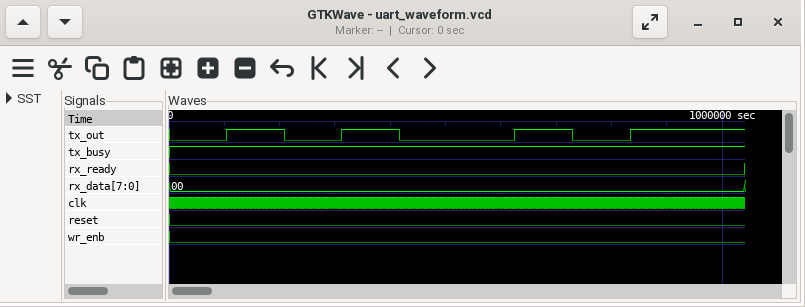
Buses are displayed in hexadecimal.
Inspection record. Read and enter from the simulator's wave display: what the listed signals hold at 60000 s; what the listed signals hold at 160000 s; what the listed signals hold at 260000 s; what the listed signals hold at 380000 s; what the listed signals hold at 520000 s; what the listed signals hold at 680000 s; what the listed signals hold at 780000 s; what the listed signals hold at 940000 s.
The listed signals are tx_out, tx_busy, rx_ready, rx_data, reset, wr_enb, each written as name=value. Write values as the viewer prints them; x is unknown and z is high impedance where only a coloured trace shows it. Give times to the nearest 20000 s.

tx_out=0, tx_busy=1, rx_ready=0, rx_data=00, reset=0, wr_enb=0
tx_out=1, tx_busy=1, rx_ready=0, rx_data=00, reset=0, wr_enb=0
tx_out=0, tx_busy=1, rx_ready=0, rx_data=00, reset=0, wr_enb=0
tx_out=1, tx_busy=1, rx_ready=0, rx_data=00, reset=0, wr_enb=0
tx_out=0, tx_busy=1, rx_ready=0, rx_data=00, reset=0, wr_enb=0
tx_out=1, tx_busy=1, rx_ready=0, rx_data=00, reset=0, wr_enb=0
tx_out=0, tx_busy=1, rx_ready=0, rx_data=00, reset=0, wr_enb=0
tx_out=1, tx_busy=1, rx_ready=0, rx_data=00, reset=0, wr_enb=0
